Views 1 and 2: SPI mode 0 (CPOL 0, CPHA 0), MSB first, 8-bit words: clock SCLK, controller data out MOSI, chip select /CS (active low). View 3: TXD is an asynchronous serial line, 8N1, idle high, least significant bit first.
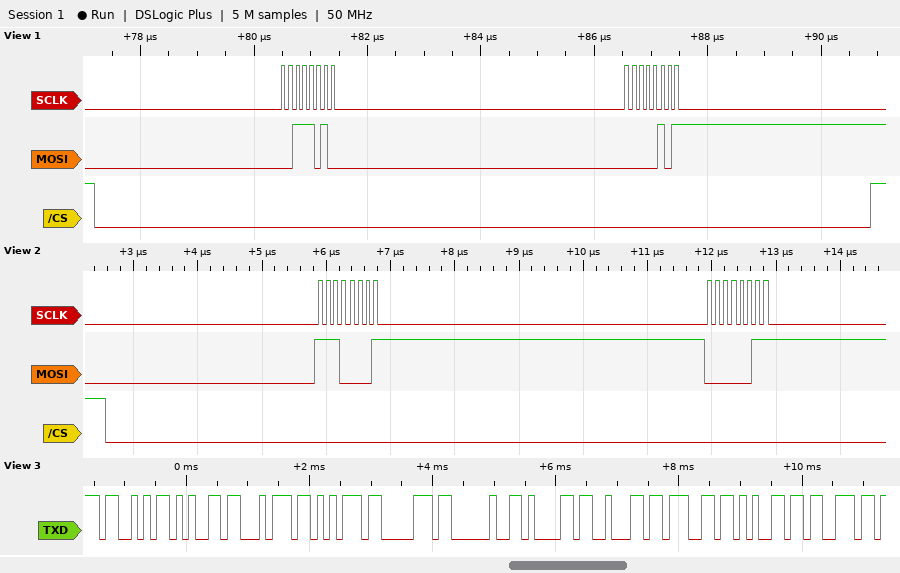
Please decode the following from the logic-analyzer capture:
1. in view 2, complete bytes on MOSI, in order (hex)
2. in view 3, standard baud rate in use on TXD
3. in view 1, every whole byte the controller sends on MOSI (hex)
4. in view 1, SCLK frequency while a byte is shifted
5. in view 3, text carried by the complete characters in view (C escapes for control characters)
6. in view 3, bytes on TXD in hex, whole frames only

E1 03
9600 baud
3A 05
8 MHz
"Setup abges"
0x53 0x65 0x74 0x75 0x70 0x20 0x61 0x62 0x67 0x65 0x73
